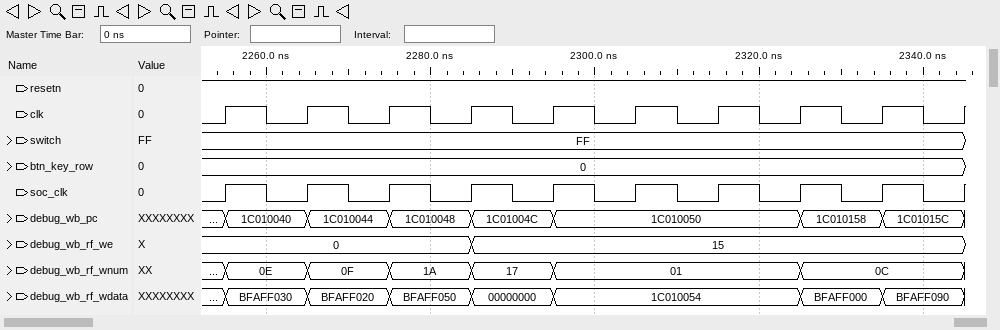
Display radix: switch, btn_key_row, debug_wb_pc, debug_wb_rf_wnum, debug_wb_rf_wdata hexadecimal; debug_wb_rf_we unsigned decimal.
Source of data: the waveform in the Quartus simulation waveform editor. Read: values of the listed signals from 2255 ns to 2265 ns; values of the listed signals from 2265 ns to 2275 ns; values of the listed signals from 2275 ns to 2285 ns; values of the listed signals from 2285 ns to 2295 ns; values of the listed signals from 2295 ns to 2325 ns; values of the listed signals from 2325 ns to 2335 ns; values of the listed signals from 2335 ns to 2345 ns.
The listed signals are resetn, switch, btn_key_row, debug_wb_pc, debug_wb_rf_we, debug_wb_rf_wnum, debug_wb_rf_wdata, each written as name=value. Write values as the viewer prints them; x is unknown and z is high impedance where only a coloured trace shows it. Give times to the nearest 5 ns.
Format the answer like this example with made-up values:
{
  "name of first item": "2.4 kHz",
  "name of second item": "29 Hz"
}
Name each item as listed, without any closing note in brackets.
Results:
{
  "values of the listed signals from 2255 ns to 2265 ns": "resetn=1, switch=FF, btn_key_row=0, debug_wb_pc=1C010040, debug_wb_rf_we=0, debug_wb_rf_wnum=0E, debug_wb_rf_wdata=BFAFF030",
  "values of the listed signals from 2265 ns to 2275 ns": "resetn=1, switch=FF, btn_key_row=0, debug_wb_pc=1C010044, debug_wb_rf_we=0, debug_wb_rf_wnum=0F, debug_wb_rf_wdata=BFAFF020",
  "values of the listed signals from 2275 ns to 2285 ns": "resetn=1, switch=FF, btn_key_row=0, debug_wb_pc=1C010048, debug_wb_rf_we=0, debug_wb_rf_wnum=1A, debug_wb_rf_wdata=BFAFF050",
  "values of the listed signals from 2285 ns to 2295 ns": "resetn=1, switch=FF, btn_key_row=0, debug_wb_pc=1C01004C, debug_wb_rf_we=15, debug_wb_rf_wnum=17, debug_wb_rf_wdata=00000000",
  "values of the listed signals from 2295 ns to 2325 ns": "resetn=1, switch=FF, btn_key_row=0, debug_wb_pc=1C010050, debug_wb_rf_we=15, debug_wb_rf_wnum=01, debug_wb_rf_wdata=1C010054",
  "values of the listed signals from 2325 ns to 2335 ns": "resetn=1, switch=FF, btn_key_row=0, debug_wb_pc=1C010158, debug_wb_rf_we=15, debug_wb_rf_wnum=0C, debug_wb_rf_wdata=BFAFF000",
  "values of the listed signals from 2335 ns to 2345 ns": "resetn=1, switch=FF, btn_key_row=0, debug_wb_pc=1C01015C, debug_wb_rf_we=15, debug_wb_rf_wnum=0C, debug_wb_rf_wdata=BFAFF090"
}
